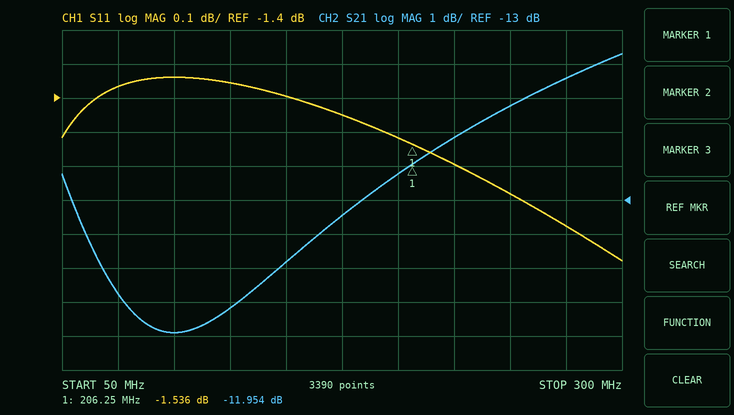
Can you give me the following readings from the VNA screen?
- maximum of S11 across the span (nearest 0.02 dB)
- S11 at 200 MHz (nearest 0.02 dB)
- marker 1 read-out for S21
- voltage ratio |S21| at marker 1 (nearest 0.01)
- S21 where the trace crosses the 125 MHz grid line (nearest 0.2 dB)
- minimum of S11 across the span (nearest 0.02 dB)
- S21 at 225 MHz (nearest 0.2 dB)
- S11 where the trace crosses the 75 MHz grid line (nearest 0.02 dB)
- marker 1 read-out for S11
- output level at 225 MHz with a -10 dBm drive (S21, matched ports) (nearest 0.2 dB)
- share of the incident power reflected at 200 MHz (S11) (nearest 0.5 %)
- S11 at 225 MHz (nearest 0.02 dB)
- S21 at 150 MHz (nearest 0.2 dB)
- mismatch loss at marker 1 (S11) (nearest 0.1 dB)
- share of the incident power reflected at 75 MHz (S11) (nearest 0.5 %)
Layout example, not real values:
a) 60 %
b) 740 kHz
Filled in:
a) -1.34 dB
b) -1.52 dB
c) -11.954 dB
d) 0.25
e) -16.2 dB
f) -1.88 dB
g) -11.2 dB
h) -1.36 dB
i) -1.536 dB
j) -21.2 dBm
k) 70.5 %
l) -1.60 dB
m) -14.8 dB
n) 5.3 dB
o) 73.0 %
